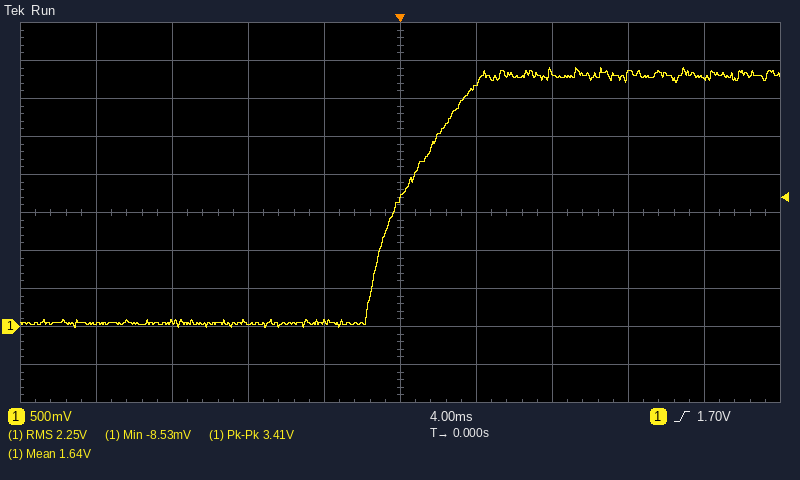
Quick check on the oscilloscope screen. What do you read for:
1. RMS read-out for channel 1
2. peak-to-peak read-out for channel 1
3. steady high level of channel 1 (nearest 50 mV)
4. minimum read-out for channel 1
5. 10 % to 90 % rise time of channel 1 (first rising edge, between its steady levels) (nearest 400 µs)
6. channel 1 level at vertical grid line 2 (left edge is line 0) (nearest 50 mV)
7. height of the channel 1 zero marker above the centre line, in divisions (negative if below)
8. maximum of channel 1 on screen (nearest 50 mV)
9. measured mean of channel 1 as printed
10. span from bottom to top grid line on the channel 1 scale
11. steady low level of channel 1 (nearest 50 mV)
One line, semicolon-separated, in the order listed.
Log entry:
2.25 V; 3.41 V; 3.30 V; -8.53 mV; 4.8 ms; 50 mV; -3.0 div; 3.40 V; 1.64 V; 5 V; 50 mV
